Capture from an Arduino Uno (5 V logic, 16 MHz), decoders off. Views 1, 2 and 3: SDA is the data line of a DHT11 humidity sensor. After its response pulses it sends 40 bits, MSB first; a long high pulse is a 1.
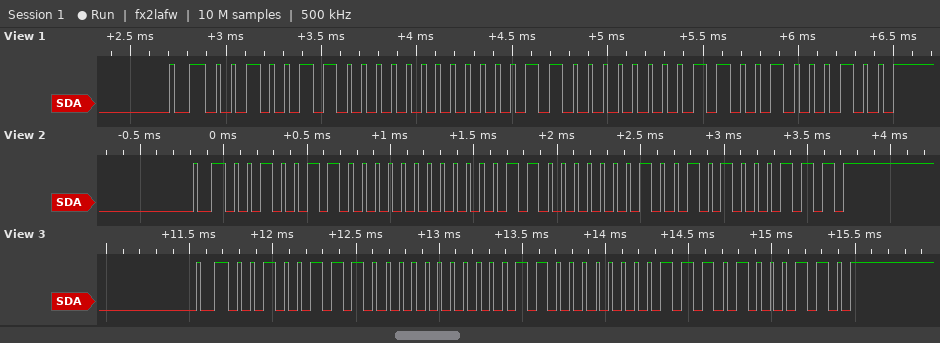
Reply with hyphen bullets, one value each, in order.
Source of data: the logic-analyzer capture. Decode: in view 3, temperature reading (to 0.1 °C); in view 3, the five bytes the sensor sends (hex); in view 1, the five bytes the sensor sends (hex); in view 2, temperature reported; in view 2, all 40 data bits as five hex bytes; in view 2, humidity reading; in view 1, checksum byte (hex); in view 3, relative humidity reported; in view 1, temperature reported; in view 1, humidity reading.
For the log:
- 24.7 °C
- 27 00 18 07 46
- 26 00 18 06 44
- 24.9 °C
- 26 00 18 09 47
- 38 %
- 0x44
- 39 %
- 24.6 °C
- 38 %
